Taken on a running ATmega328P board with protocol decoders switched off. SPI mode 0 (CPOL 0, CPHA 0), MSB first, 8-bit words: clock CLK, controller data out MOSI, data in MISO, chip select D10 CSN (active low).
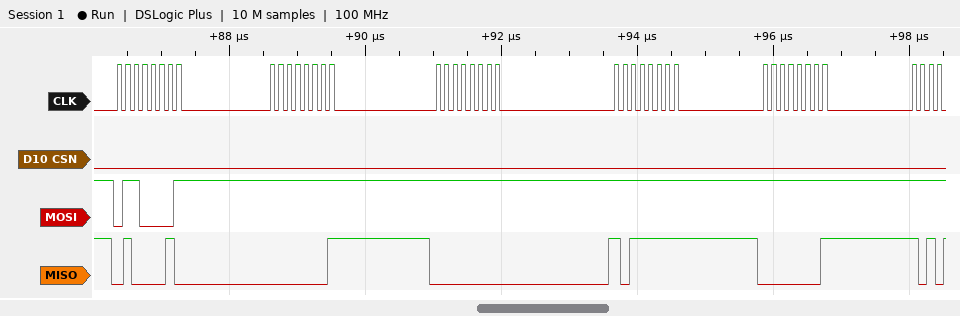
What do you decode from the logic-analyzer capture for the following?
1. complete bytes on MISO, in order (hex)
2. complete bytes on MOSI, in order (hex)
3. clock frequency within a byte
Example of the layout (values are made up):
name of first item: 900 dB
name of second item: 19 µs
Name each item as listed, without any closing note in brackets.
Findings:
complete bytes on MISO, in order: 42 01 00 BF 01
complete bytes on MOSI, in order: 61 FF FF FF FF
clock frequency within a byte: 8 MHz
